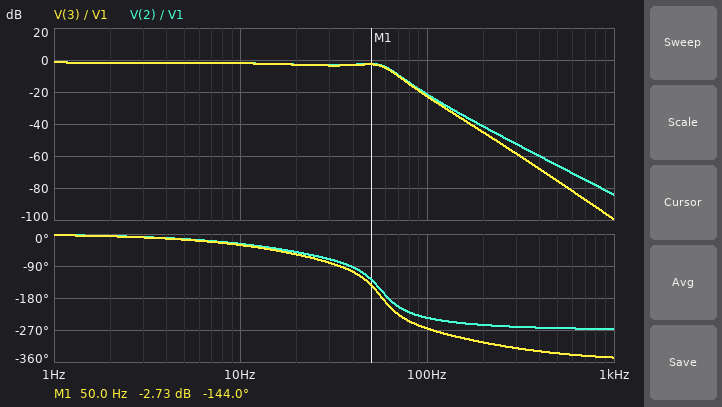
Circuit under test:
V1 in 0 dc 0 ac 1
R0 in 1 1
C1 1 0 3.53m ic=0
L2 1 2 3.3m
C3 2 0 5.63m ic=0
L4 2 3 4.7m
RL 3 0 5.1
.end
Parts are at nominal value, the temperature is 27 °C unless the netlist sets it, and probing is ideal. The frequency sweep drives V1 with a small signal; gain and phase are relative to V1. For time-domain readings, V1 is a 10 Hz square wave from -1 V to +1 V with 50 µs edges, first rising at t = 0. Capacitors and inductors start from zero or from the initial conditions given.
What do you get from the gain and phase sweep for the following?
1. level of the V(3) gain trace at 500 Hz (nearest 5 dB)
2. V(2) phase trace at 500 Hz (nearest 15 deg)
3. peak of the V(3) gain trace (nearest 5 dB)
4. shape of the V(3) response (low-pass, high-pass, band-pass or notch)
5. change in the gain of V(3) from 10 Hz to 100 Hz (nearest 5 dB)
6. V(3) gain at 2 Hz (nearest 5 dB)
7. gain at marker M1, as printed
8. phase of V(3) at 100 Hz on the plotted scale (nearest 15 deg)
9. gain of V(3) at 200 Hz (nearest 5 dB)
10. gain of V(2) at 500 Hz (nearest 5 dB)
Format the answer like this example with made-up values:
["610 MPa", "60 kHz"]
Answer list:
["-75 dB", "-270 deg", "0 dB", "low-pass", "-20 dB", "0 dB", "-2.73 dB", "-270 deg", "-45 dB", "-65 dB"]
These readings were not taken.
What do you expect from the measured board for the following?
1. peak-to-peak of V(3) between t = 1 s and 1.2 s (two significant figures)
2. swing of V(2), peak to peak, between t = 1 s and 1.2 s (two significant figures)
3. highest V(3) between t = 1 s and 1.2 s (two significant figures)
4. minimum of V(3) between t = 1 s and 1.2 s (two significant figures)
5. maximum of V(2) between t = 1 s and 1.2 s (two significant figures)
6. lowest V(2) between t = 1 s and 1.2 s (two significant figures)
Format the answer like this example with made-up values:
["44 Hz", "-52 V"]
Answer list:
["1.7 V", "1.7 V", "870 mV", "-870 mV", "870 mV", "-870 mV"]
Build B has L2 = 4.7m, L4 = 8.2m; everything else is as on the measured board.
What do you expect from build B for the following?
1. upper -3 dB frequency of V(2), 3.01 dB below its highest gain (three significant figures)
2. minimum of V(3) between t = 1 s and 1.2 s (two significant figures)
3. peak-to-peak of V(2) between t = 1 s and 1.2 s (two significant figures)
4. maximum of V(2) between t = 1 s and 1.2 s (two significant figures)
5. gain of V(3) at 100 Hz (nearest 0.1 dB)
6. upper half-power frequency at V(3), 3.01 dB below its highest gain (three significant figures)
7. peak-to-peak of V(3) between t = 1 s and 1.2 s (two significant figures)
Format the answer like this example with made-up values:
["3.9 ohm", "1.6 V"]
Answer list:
["50.6 Hz", "-950 mV", "2.0 V", "980 mV", "-28.7 dB", "48.8 Hz", "1.9 V"]
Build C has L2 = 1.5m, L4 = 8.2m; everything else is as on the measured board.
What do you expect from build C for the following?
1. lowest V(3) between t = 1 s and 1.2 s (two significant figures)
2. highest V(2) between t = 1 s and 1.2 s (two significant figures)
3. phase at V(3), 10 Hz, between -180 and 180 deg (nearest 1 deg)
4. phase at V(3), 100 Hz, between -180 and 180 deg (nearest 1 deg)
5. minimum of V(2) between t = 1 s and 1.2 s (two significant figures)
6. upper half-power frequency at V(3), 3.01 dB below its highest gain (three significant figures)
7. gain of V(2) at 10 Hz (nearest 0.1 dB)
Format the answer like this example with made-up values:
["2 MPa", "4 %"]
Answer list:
["-840 mV", "850 mV", "-32 deg", "103 deg", "-850 mV", "25.0 Hz", "-2.2 dB"]
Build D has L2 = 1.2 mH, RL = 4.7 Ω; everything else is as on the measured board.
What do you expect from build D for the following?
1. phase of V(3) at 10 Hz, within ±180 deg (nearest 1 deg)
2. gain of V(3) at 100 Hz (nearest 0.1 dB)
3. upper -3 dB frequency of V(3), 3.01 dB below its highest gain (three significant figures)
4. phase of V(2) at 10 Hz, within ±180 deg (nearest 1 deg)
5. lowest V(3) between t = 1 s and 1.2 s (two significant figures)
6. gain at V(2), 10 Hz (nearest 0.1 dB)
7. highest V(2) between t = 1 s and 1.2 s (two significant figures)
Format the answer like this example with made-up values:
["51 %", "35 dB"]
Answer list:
["-29 deg", "-6.0 dB", "24.8 Hz", "-26 deg", "-830 mV", "-2.4 dB", "830 mV"]
